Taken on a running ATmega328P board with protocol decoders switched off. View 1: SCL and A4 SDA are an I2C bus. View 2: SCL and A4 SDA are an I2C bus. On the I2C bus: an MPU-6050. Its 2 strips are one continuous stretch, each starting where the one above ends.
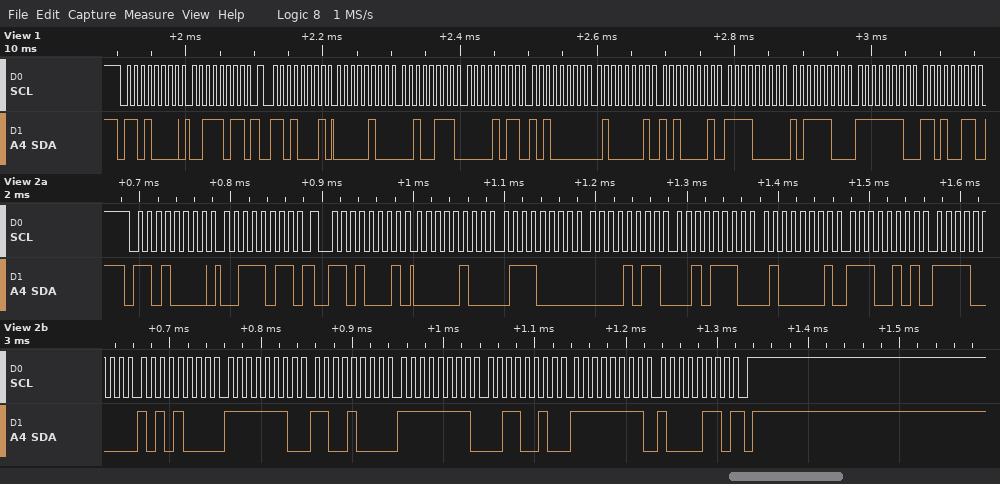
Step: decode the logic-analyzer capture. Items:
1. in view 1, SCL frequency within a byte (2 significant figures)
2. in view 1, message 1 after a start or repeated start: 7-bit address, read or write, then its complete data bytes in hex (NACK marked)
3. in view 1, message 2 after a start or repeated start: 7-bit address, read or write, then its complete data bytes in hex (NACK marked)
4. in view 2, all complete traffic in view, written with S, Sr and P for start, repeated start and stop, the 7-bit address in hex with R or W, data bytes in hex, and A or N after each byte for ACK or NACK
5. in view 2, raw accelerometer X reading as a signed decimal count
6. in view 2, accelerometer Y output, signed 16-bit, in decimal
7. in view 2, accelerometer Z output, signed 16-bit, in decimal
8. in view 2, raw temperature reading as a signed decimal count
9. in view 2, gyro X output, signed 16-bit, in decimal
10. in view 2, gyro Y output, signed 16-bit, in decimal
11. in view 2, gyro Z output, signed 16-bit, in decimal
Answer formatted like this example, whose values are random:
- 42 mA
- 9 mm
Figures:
- 100 kHz
- 0x68 write: 3B
- 0x68 read: 04 27 0B A0 41 A1 F0 BC FE D3
- S 68W A 3B A Sr 68R A 04 A 70 A 0B A 2E A 41 A E5 A F0 A A8 A FE A C8 A FF A 32 A FF A 86 N P
- 1136
- 2862
- 16869
- -3928
- -312
- -206
- -122
